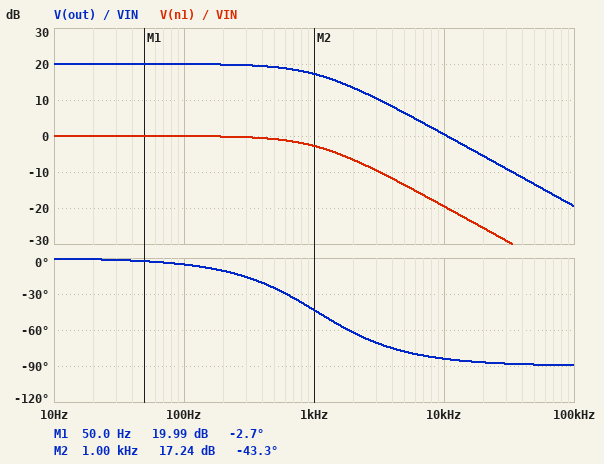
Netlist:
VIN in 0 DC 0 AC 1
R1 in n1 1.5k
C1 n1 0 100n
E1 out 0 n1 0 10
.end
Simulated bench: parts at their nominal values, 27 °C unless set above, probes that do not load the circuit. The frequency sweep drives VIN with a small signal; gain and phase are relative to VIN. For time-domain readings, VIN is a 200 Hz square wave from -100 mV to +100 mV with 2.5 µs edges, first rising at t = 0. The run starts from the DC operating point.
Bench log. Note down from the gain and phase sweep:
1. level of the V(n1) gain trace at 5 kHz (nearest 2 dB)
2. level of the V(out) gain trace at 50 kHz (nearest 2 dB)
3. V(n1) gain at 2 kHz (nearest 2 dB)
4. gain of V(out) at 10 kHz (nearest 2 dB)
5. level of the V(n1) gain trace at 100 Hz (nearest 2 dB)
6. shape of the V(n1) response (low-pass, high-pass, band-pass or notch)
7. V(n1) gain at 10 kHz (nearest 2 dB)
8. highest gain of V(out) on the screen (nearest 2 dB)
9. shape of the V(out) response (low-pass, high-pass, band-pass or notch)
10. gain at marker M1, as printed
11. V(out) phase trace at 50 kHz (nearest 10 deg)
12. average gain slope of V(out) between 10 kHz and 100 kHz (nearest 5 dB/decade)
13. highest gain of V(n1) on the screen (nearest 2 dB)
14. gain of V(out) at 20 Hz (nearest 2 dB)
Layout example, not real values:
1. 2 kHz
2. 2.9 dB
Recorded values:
1. -14 dB
2. -14 dB
3. -6 dB
4. 0 dB
5. 0 dB
6. low-pass
7. -20 dB
8. 20 dB
9. low-pass
10. 19.99 dB
11. -90 deg
12. -20 dB/decade
13. 0 dB
14. 20 dB
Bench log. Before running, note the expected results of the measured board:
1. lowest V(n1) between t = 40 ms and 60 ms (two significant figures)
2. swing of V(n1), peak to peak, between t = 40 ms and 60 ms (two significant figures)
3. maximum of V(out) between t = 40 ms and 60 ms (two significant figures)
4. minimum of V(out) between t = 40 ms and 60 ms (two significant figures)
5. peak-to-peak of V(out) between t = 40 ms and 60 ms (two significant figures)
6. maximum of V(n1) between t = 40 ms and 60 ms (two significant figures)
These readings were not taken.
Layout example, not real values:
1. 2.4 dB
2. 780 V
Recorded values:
1. -100 mV
2. 200 mV
3. 1.0 V
4. -1.0 V
5. 2.0 V
6. 100 mV
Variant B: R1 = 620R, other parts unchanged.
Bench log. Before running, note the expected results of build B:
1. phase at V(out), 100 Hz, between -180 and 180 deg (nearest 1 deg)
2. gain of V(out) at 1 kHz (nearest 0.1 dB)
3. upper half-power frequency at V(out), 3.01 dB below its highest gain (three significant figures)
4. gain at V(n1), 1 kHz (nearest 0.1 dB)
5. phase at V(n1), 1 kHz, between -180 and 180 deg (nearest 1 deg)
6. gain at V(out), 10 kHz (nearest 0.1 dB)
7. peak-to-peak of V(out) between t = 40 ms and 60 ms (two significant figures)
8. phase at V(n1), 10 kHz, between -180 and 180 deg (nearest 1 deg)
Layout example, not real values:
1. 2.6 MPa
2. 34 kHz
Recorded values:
1. -2 deg
2. 19.4 dB
3. 2.57 kHz
4. -0.6 dB
5. -21 deg
6. 7.9 dB
7. 2.0 V
8. -76 deg
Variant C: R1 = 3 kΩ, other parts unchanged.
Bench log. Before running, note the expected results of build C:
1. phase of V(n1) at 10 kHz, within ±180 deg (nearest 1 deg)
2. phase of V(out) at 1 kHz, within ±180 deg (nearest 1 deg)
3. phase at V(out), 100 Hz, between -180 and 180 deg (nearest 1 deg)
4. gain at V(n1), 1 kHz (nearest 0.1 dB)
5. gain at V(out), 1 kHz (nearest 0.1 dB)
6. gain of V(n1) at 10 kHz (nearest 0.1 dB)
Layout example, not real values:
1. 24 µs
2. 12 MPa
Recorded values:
1. -87 deg
2. -62 deg
3. -11 deg
4. -6.6 dB
5. 13.4 dB
6. -25.5 dB
